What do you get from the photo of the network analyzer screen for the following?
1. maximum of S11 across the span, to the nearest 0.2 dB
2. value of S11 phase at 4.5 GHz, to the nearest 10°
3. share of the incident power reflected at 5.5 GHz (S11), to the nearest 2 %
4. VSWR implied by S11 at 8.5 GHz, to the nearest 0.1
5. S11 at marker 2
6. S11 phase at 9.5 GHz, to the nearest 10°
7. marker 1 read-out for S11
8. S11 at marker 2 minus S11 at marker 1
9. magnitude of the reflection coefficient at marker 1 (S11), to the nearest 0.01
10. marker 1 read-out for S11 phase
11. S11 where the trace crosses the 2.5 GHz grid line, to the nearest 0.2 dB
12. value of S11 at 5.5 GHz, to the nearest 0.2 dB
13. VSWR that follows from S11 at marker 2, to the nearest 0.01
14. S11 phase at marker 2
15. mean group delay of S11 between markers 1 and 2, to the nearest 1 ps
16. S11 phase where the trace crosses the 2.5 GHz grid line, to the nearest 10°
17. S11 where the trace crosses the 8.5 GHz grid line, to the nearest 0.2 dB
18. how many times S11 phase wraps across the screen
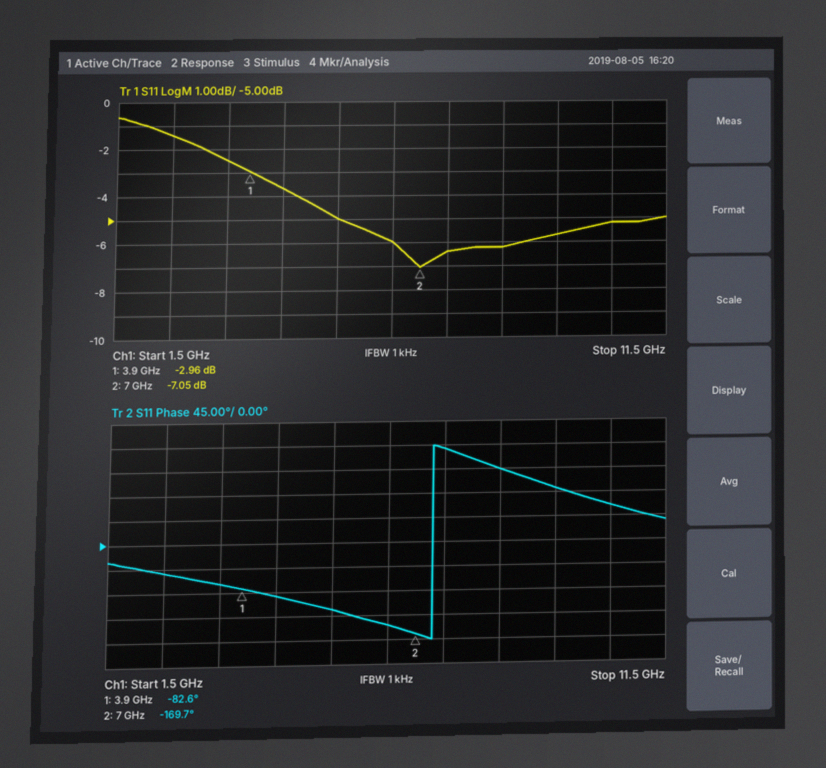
-0.6 dB
-100°
32 %
2.9
-7.05 dB
100°
-2.96 dB
-4.09 dB
0.71
-82.6°
-1.4 dB
-5.0 dB
2.60
-169.7°
78 ps
-50°
-6.2 dB
1
